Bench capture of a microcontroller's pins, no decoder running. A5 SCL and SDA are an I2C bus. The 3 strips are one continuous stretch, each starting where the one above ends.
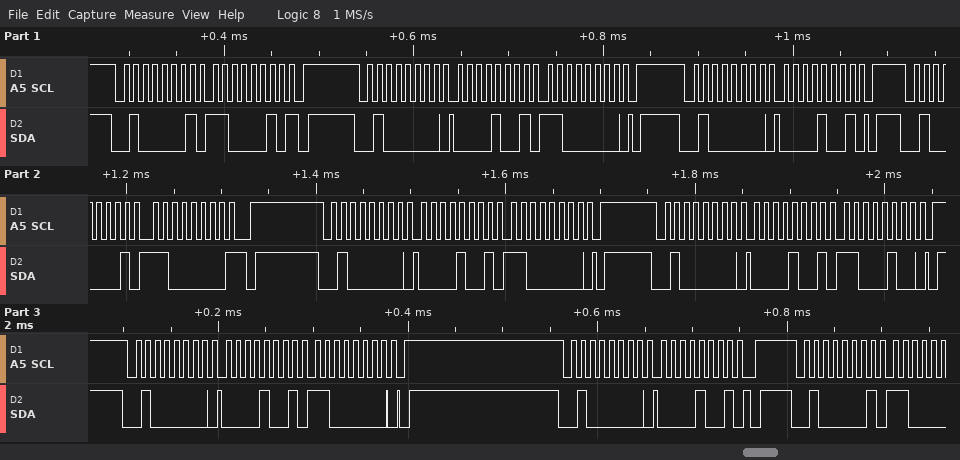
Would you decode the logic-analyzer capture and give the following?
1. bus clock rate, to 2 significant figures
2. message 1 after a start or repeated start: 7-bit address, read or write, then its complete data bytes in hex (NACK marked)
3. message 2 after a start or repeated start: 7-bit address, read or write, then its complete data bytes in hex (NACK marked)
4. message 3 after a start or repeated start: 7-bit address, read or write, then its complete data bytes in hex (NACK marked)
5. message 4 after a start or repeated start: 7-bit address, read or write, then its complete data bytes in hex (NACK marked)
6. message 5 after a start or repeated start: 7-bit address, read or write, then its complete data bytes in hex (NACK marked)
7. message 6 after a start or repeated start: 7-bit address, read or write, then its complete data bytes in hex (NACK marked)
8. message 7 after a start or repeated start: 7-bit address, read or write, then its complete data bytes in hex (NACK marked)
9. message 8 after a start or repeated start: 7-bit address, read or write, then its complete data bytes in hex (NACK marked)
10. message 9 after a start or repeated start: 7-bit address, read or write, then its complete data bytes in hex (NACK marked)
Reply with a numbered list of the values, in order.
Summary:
1. 100 kHz
2. 0x20 read: C2 NACK
3. 0x20 write: 09 C0
4. 0x20 write: 09
5. 0x20 read: C0 NACK
6. 0x20 write: 09 C0
7. 0x20 write: 09 C4
8. 0x20 write: 09 C0
9. 0x20 write: 09
10. 0x20 read
